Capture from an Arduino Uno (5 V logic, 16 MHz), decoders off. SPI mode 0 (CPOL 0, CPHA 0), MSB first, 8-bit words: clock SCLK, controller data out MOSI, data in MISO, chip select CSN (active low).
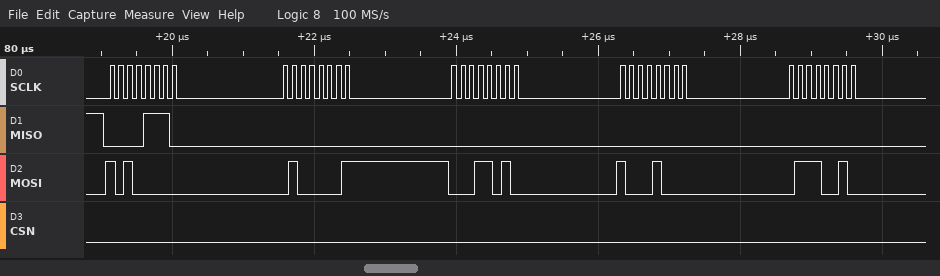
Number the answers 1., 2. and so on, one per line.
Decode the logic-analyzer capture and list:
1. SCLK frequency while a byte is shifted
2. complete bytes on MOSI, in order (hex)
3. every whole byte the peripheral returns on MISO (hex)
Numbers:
1. 8 MHz
2. A0 41 1A 88 72
3. 0E 00 00 00 00
